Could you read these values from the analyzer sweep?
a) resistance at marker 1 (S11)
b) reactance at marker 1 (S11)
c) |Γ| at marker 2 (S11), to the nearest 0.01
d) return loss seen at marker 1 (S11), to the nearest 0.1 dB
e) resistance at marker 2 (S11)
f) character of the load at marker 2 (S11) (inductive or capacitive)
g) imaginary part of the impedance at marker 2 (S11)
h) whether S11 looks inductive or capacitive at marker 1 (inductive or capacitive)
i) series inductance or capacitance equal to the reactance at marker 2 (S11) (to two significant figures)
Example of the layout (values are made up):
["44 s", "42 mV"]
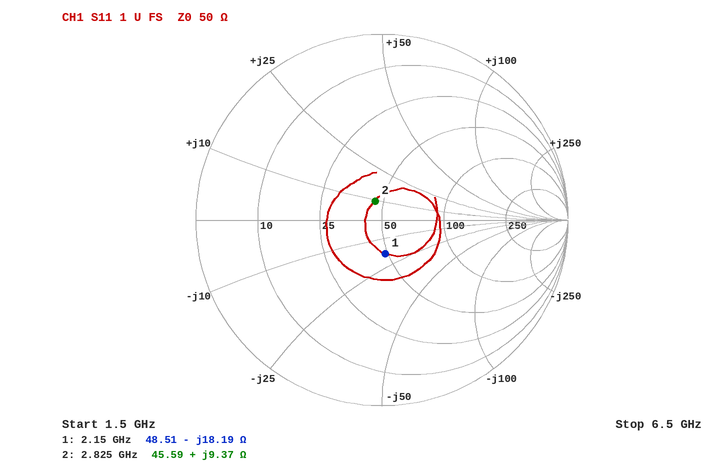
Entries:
["48.51 Ω", "-18.19 Ω", "0.11", "14.8 dB", "45.59 Ω", "inductive", "+9.37 Ω", "capacitive", "530 pH"]
